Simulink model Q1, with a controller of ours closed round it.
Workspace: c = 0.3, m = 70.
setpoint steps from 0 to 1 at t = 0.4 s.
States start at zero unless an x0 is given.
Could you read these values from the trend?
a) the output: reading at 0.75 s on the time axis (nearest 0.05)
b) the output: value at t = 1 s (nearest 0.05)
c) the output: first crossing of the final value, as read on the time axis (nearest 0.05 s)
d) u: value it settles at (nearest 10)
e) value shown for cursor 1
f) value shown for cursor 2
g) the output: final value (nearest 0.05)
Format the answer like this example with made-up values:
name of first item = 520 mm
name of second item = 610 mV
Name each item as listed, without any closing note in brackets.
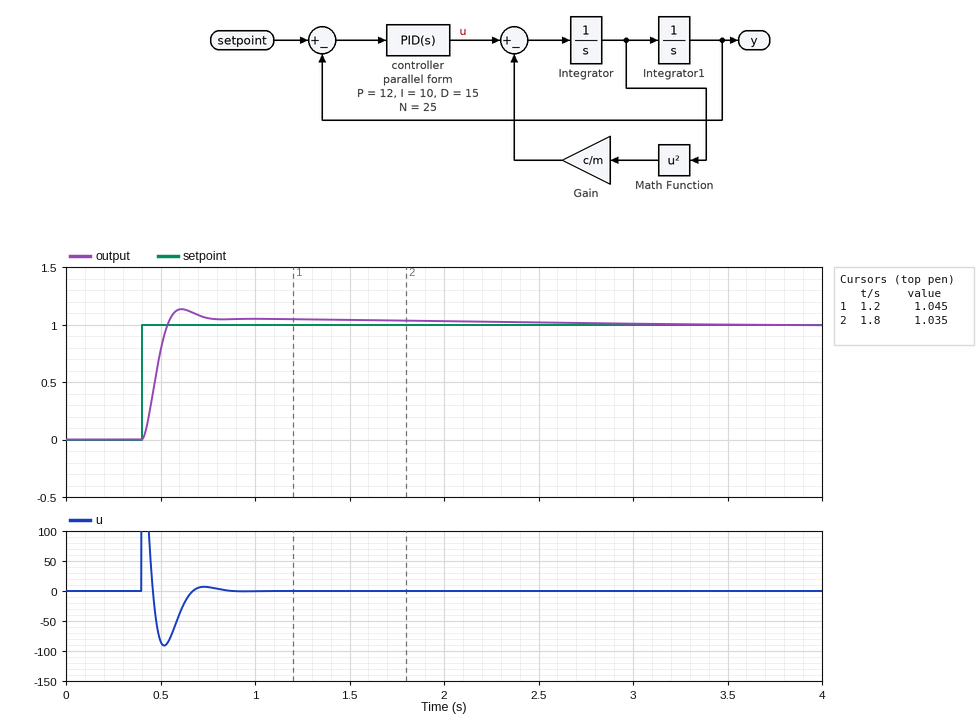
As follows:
the output: reading at 0.75 s on the time axis = 1.05
the output: value at t = 1 s = 1.05
the output: first crossing of the final value, as read on the time axis = 0.55 s
u: value it settles at = 0
value shown for cursor 1 = 1.045
value shown for cursor 2 = 1.035
the output: final value = 1.00
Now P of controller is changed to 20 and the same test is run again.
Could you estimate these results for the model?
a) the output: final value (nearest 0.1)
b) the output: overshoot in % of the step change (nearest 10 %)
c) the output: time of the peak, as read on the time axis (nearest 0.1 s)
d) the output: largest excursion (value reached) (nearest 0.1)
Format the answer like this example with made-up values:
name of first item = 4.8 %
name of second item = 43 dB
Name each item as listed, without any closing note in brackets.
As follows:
the output: final value = 1.0
the output: overshoot in % of the step change = 20 %
the output: time of the peak, as read on the time axis = 0.6 s
the output: largest excursion (value reached) = 1.2
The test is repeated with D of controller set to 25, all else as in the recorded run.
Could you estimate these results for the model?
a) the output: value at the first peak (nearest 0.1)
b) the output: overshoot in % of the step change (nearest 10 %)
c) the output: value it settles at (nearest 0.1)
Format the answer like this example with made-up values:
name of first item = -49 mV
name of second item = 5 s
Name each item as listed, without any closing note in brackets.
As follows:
the output: value at the first peak = 1.2
the output: overshoot in % of the step change = 20 %
the output: value it settles at = 1.0
